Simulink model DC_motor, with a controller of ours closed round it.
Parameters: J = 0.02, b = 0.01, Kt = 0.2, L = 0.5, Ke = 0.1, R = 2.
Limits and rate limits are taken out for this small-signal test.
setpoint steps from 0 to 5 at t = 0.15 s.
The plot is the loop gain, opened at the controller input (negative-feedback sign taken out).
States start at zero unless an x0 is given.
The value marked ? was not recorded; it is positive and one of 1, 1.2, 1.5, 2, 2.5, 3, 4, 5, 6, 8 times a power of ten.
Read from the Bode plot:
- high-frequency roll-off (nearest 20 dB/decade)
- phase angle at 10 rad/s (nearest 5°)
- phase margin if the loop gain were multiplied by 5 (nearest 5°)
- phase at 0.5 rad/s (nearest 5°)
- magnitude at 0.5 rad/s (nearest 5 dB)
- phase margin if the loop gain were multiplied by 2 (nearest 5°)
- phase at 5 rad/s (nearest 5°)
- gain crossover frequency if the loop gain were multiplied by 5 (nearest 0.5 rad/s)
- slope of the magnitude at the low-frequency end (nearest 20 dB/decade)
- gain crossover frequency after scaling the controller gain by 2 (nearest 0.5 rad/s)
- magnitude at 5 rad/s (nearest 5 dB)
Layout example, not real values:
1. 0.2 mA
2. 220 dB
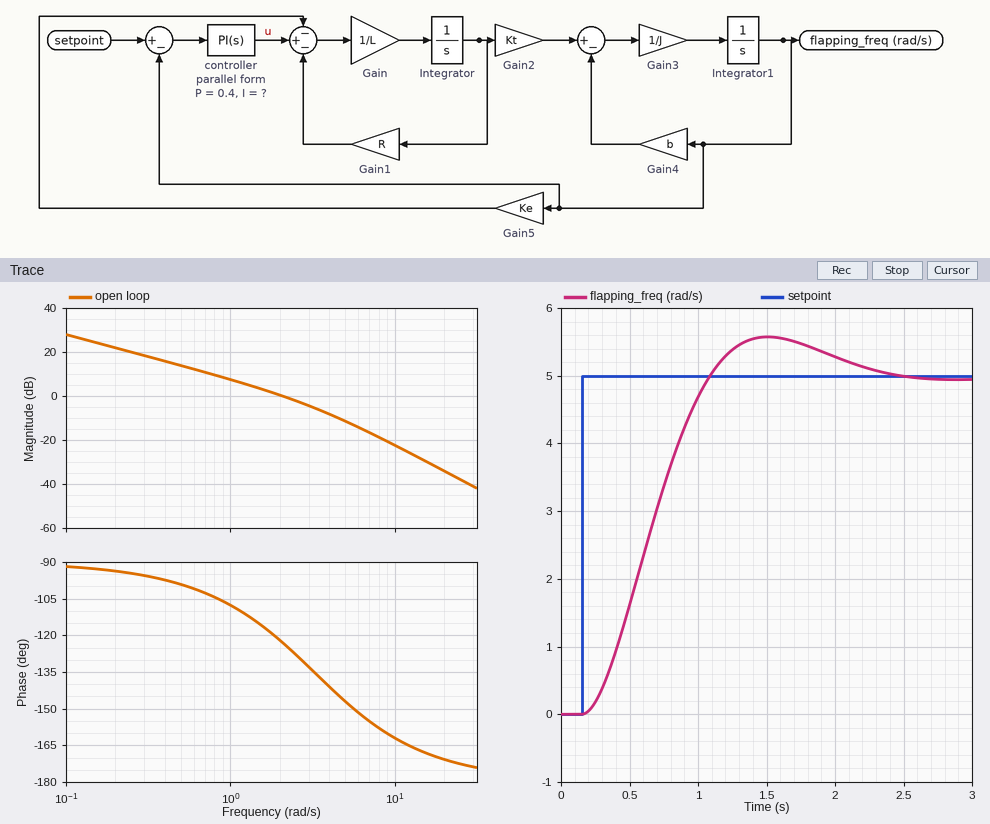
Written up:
1. -40 dB/decade
2. -160°
3. 30°
4. -100°
5. 15 dB
6. 45°
7. -145°
8. 6.0 rad/s
9. -20 dB/decade
10. 3.5 rad/s
11. -10 dB
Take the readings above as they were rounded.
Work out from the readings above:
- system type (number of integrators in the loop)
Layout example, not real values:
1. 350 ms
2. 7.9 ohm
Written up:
1. 1
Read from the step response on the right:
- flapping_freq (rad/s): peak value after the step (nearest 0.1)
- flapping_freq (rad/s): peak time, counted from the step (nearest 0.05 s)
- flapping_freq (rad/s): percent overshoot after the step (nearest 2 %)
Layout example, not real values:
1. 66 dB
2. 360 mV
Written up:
1. 5.6
2. 1.35 s
3. 12 %
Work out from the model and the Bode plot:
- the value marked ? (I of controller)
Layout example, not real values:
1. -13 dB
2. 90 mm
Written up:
1. 0.5
